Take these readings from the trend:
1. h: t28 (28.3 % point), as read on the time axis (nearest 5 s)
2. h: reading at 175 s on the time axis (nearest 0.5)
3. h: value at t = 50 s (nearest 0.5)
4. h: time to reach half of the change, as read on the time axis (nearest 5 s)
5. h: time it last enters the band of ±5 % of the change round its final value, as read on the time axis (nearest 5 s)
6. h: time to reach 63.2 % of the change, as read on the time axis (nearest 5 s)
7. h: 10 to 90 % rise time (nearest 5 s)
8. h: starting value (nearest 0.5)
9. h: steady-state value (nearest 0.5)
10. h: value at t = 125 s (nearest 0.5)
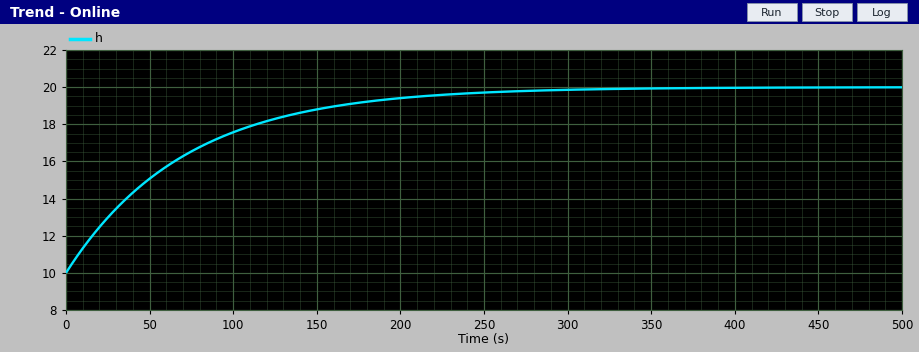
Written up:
25 s
19.0
15.0
50 s
210 s
70 s
155 s
10.0
20.0
18.5
